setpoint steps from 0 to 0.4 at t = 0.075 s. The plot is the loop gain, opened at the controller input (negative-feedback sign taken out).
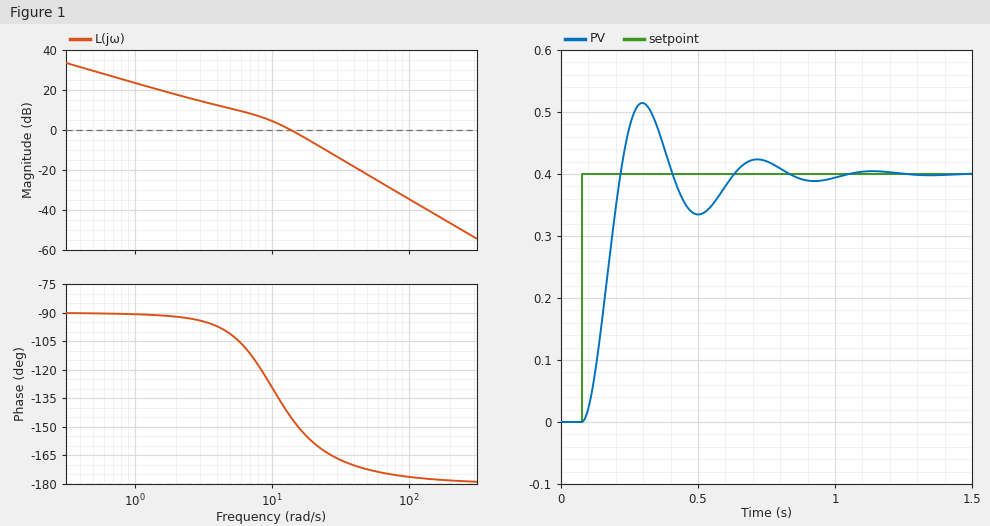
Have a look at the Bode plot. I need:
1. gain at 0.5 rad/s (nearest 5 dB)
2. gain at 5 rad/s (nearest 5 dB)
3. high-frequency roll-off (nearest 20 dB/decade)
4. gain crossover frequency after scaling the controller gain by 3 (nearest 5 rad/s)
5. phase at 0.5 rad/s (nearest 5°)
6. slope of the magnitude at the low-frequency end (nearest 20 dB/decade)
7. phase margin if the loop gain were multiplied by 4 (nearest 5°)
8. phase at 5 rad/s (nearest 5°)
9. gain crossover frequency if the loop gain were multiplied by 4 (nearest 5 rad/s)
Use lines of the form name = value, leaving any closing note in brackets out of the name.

gain at 0.5 rad/s = 30 dB
gain at 5 rad/s = 10 dB
high-frequency roll-off = -40 dB/decade
gain crossover frequency after scaling the controller gain by 3 = 25 rad/s
phase at 0.5 rad/s = -90°
slope of the magnitude at the low-frequency end = -20 dB/decade
phase margin if the loop gain were multiplied by 4 = 15°
phase at 5 rad/s = -100°
gain crossover frequency if the loop gain were multiplied by 4 = 30 rad/s
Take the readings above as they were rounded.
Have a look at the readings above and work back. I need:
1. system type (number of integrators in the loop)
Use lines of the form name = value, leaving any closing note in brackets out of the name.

system type = 1
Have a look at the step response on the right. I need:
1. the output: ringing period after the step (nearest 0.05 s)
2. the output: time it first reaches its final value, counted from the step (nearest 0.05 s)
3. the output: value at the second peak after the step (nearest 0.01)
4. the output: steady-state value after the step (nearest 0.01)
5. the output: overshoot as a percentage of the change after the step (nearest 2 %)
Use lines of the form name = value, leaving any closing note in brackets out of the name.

the output: ringing period after the step = 0.40 s
the output: time it first reaches its final value, counted from the step = 0.15 s
the output: value at the second peak after the step = 0.42
the output: steady-state value after the step = 0.40
the output: overshoot as a percentage of the change after the step = 28 %
